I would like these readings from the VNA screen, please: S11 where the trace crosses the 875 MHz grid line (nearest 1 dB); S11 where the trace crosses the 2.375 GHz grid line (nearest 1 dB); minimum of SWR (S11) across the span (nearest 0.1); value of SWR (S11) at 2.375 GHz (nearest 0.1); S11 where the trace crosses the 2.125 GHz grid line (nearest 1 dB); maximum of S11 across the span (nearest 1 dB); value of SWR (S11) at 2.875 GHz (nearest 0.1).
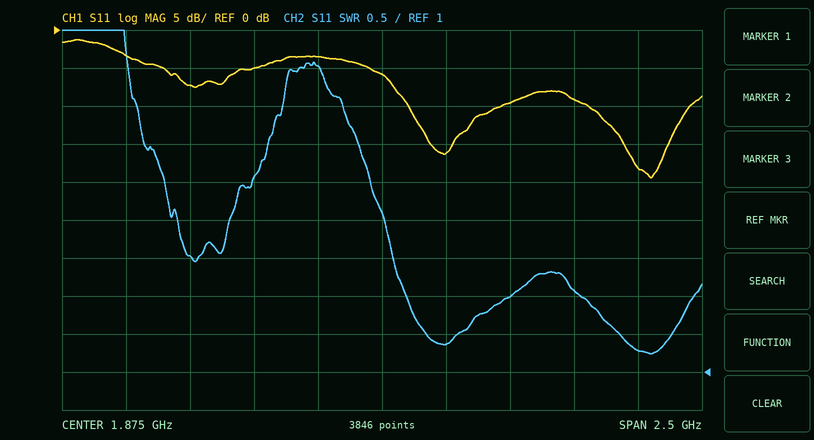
-3 dB
-10 dB
1.2
2.0
-16 dB
-1 dB
1.3
